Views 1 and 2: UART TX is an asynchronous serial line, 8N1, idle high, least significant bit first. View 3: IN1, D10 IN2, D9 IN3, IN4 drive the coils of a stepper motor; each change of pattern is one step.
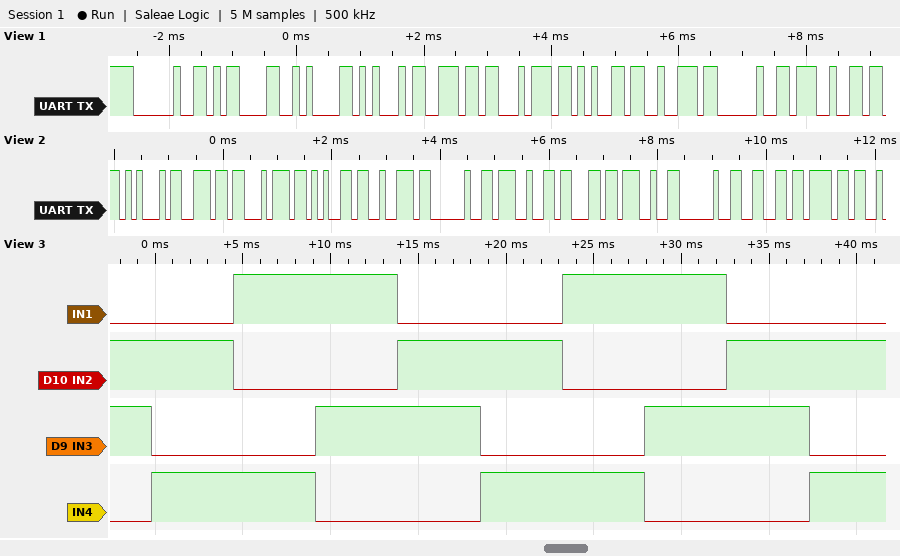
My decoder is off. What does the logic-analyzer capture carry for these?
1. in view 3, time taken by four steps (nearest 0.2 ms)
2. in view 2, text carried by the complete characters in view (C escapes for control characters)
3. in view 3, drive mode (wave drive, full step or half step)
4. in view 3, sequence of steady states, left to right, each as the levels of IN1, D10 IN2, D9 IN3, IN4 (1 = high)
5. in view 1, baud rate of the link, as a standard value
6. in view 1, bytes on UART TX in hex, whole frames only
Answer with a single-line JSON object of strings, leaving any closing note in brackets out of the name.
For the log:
{"in view 3, time taken by four steps": "18.8 ms", "in view 2, text carried by the complete characters in view": "\"Enter 'c' fo\"", "in view 3, drive mode": "full step", "in view 3, sequence of steady states, left to right, each as the levels of IN1, D10 IN2, D9 IN3, IN4": "0110 0101 1001 1010 0110 0101 1001 1010 0110 0101", "in view 1, baud rate of the link, as a standard value": "9600 baud", "in view 1, bytes on UART TX in hex, whole frames only": "20 0D 0A 45 6E 74 65 72 20 27"}
